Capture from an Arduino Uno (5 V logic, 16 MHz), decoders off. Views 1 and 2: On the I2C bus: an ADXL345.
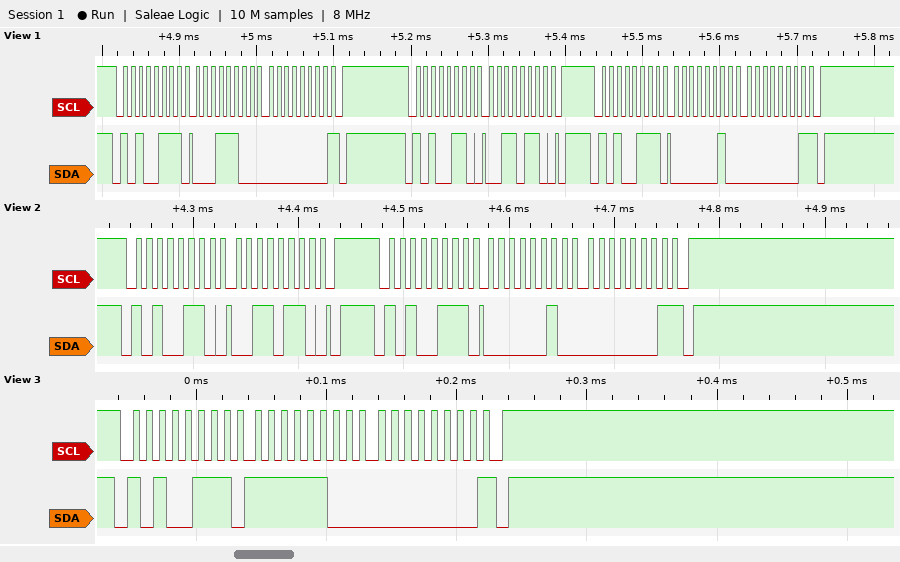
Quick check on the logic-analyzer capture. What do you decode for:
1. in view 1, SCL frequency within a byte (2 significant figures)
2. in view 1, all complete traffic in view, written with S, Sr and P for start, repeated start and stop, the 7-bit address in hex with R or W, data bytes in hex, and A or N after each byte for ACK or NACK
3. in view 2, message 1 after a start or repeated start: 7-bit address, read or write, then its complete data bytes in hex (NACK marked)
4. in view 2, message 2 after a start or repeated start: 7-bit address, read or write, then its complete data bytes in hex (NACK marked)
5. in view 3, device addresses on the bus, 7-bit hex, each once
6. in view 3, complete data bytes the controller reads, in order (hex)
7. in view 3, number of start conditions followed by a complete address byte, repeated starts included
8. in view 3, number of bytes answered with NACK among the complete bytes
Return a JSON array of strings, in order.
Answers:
["100 kHz", "S 53R A 1C A 00 N P S 53W A 36 A P S 53R A 02 A 01 N P", "0x53 write: 36", "0x53 read: 02 01 NACK", "0x53", "FC 00", "1", "1"]
